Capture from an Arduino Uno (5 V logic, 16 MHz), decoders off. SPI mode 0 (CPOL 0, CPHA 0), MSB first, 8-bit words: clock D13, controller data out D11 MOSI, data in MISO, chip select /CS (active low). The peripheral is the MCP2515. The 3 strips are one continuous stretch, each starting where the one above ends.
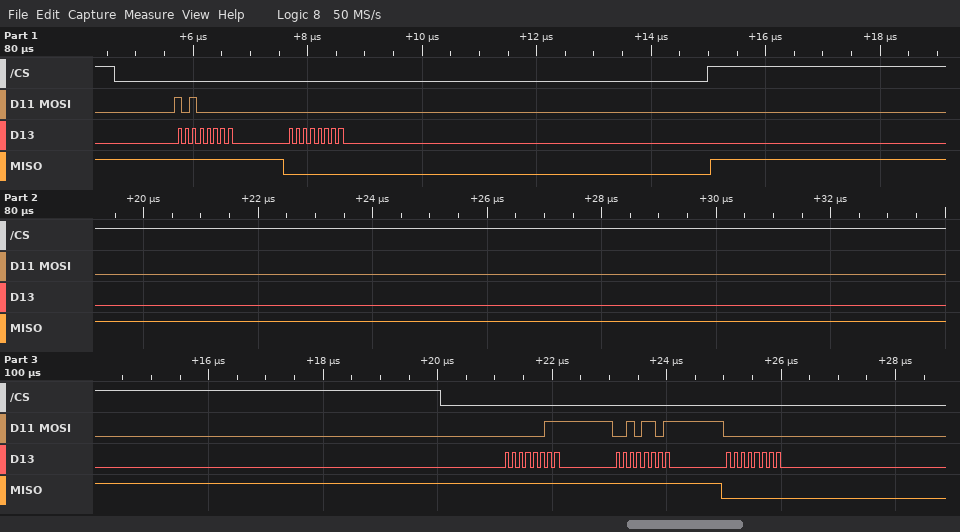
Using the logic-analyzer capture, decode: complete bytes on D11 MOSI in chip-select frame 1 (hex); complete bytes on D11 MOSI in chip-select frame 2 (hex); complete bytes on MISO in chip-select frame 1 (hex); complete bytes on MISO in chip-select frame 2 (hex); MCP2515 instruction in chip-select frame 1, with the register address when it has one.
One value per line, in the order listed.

A0 00
03 2D 00
FF 00
FF FF 00
READ STATUS
